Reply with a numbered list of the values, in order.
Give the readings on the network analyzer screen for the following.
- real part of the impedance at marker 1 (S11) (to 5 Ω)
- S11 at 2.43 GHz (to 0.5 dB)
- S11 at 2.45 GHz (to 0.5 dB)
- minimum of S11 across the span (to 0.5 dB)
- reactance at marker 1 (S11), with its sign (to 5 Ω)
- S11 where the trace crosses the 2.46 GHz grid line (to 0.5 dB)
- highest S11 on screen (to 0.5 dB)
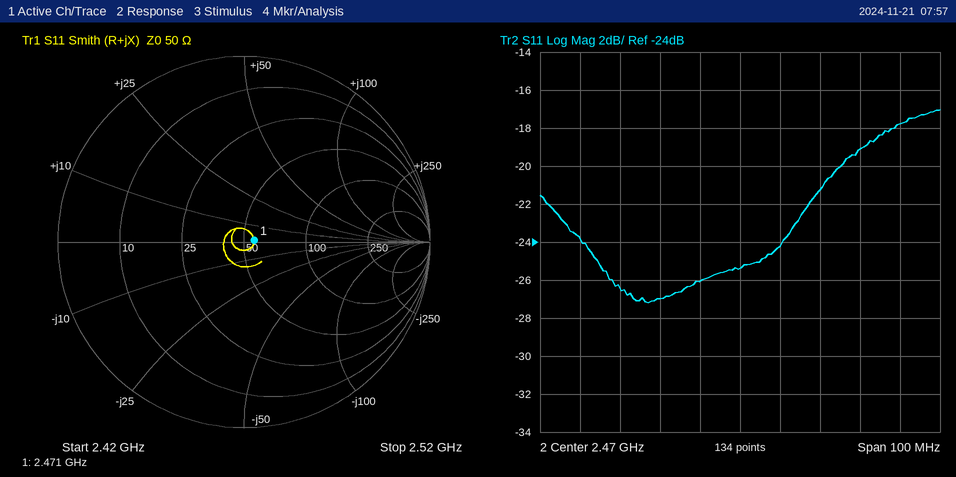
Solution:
1. 55 Ω
2. -24.0 dB
3. -27.0 dB
4. -27.0 dB
5. 0 Ω
6. -26.0 dB
7. -17.0 dB
